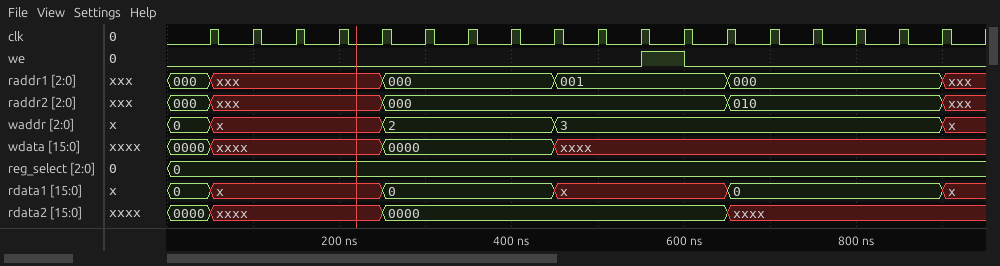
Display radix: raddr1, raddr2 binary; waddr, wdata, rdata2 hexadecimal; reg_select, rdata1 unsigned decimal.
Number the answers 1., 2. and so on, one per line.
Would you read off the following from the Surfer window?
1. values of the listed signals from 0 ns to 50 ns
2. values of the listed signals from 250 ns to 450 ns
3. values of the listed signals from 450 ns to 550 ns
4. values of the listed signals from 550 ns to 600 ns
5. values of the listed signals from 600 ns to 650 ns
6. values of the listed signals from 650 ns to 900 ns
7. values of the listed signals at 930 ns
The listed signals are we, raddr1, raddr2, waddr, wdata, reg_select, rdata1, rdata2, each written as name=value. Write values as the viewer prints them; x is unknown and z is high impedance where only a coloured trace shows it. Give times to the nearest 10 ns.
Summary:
1. we=0, raddr1=000, raddr2=000, waddr=0, wdata=0000, reg_select=0, rdata1=0, rdata2=0000
2. we=0, raddr1=000, raddr2=000, waddr=2, wdata=0000, reg_select=0, rdata1=0, rdata2=0000
3. we=0, raddr1=001, raddr2=000, waddr=3, wdata=xxxx, reg_select=0, rdata1=x, rdata2=0000
4. we=1, raddr1=001, raddr2=000, waddr=3, wdata=xxxx, reg_select=0, rdata1=x, rdata2=0000
5. we=0, raddr1=001, raddr2=000, waddr=3, wdata=xxxx, reg_select=0, rdata1=x, rdata2=0000
6. we=0, raddr1=000, raddr2=010, waddr=3, wdata=xxxx, reg_select=0, rdata1=0, rdata2=xxxx
7. we=0, raddr1=xxx, raddr2=xxx, waddr=x, wdata=xxxx, reg_select=0, rdata1=x, rdata2=xxxx
